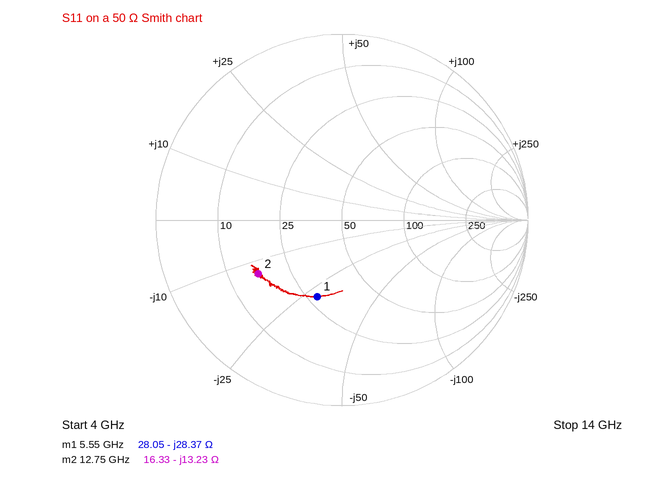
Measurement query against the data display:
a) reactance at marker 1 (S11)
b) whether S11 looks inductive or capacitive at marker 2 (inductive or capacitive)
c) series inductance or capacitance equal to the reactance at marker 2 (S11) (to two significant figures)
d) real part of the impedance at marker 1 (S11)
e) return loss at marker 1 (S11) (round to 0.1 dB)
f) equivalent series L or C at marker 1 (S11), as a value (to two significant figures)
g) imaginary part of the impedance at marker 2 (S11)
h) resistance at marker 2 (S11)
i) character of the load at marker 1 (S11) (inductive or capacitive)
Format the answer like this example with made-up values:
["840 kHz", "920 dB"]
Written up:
["-28.37 Ω", "capacitive", "940 fF", "28.05 Ω", "7.3 dB", "1.0 pF", "-13.23 Ω", "16.33 Ω", "capacitive"]
